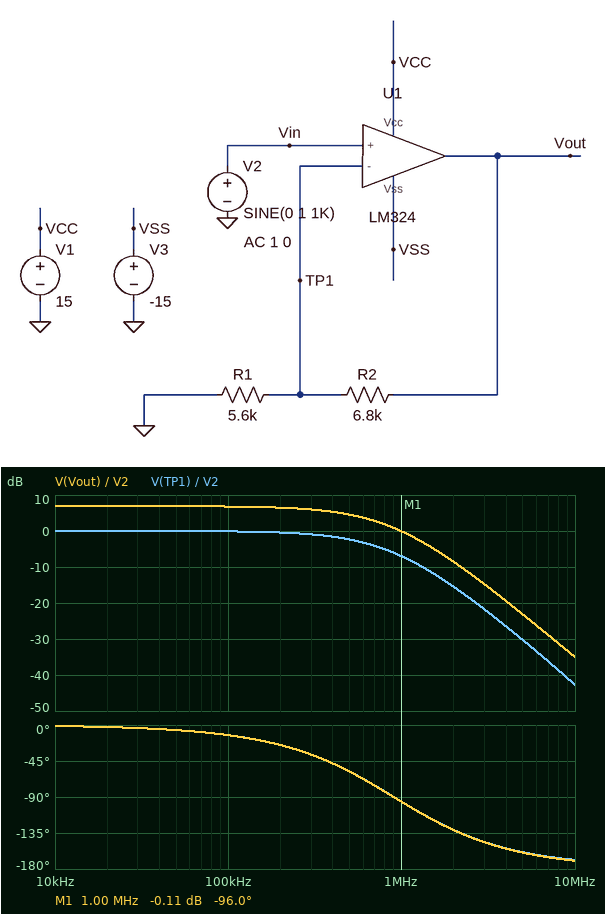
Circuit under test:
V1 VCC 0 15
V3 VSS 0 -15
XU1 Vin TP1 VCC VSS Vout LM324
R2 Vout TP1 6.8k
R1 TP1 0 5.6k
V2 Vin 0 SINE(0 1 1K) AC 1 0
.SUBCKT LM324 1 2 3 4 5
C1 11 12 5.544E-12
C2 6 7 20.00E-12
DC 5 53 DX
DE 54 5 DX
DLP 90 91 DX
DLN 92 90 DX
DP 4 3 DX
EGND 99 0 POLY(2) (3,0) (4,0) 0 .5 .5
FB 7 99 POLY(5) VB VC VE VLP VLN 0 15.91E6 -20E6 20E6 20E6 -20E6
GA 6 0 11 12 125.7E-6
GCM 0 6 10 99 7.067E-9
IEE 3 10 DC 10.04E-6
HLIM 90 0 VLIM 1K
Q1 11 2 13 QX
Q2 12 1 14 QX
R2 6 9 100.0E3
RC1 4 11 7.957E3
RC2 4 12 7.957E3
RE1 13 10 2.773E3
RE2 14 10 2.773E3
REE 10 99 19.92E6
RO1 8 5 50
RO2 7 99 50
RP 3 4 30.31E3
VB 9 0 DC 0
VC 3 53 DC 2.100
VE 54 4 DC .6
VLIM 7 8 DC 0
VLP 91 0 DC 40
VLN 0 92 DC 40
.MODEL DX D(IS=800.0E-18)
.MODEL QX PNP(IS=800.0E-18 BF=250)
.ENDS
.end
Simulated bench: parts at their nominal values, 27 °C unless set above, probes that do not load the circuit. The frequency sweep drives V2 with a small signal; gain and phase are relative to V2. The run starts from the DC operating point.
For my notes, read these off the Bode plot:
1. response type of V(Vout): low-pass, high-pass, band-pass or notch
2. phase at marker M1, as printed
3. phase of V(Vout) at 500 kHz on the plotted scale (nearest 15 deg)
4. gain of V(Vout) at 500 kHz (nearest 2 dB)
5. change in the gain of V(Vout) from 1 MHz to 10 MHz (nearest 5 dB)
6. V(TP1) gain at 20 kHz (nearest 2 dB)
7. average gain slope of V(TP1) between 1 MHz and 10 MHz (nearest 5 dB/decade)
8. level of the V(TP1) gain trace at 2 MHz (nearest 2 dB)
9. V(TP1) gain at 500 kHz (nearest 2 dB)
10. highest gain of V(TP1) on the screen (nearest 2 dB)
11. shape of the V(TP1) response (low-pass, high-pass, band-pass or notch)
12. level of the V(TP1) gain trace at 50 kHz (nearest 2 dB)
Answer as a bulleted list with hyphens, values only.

- low-pass
- -96.0 deg
- -60 deg
- 4 dB
- -35 dB
- 0 dB
- -35 dB/decade
- -16 dB
- -2 dB
- 0 dB
- low-pass
- 0 dB
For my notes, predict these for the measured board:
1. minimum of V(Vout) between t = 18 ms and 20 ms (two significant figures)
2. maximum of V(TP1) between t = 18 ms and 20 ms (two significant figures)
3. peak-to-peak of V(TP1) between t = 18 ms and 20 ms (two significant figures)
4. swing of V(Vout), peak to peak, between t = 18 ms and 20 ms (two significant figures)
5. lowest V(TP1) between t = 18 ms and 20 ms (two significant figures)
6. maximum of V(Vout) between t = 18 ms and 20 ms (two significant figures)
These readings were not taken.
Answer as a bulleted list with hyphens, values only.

- -2.2 V
- 1.0 V
- 2.0 V
- 4.4 V
- -1.0 V
- 2.2 V
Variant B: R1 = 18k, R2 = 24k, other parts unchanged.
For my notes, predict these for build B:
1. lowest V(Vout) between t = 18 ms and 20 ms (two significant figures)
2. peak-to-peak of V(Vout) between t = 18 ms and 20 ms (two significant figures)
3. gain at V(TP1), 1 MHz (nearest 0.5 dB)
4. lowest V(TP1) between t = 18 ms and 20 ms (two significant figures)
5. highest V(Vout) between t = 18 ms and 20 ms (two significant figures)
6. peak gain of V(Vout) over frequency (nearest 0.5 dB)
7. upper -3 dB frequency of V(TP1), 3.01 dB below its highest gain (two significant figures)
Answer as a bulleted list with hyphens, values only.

- -2.3 V
- 4.7 V
- -7.5 dB
- -1.0 V
- 2.3 V
- 7.5 dB
- 540 kHz
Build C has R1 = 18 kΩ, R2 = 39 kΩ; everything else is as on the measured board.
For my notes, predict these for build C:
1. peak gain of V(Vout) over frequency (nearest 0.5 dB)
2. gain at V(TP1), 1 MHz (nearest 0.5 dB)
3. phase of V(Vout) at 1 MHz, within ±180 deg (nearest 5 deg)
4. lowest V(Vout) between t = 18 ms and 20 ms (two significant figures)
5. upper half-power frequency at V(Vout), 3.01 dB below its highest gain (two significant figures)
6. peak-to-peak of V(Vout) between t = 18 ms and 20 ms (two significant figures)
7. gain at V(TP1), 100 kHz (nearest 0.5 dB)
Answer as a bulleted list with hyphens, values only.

- 10.0 dB
- -10.5 dB
- -105 deg
- -3.2 V
- 380 kHz
- 6.3 V
- -0.5 dB
